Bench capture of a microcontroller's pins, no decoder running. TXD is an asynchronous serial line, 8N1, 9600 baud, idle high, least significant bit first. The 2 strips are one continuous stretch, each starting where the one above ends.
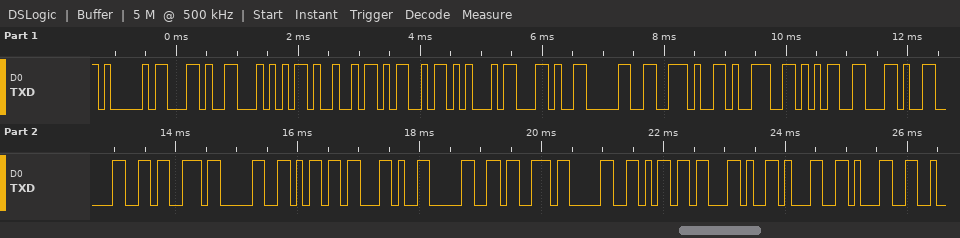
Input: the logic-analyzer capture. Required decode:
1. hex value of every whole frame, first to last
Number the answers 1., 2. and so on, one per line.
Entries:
1. 0x41 0x2C 0x54 0x49 0x4D 0x45 0x2C 0x30 0x2E 0x39 0x35 0x2C 0x30 0x73 0x30 0x6D 0x2C 0x30 0x73 0x30 0x6D 0x2C 0x31 0x31
